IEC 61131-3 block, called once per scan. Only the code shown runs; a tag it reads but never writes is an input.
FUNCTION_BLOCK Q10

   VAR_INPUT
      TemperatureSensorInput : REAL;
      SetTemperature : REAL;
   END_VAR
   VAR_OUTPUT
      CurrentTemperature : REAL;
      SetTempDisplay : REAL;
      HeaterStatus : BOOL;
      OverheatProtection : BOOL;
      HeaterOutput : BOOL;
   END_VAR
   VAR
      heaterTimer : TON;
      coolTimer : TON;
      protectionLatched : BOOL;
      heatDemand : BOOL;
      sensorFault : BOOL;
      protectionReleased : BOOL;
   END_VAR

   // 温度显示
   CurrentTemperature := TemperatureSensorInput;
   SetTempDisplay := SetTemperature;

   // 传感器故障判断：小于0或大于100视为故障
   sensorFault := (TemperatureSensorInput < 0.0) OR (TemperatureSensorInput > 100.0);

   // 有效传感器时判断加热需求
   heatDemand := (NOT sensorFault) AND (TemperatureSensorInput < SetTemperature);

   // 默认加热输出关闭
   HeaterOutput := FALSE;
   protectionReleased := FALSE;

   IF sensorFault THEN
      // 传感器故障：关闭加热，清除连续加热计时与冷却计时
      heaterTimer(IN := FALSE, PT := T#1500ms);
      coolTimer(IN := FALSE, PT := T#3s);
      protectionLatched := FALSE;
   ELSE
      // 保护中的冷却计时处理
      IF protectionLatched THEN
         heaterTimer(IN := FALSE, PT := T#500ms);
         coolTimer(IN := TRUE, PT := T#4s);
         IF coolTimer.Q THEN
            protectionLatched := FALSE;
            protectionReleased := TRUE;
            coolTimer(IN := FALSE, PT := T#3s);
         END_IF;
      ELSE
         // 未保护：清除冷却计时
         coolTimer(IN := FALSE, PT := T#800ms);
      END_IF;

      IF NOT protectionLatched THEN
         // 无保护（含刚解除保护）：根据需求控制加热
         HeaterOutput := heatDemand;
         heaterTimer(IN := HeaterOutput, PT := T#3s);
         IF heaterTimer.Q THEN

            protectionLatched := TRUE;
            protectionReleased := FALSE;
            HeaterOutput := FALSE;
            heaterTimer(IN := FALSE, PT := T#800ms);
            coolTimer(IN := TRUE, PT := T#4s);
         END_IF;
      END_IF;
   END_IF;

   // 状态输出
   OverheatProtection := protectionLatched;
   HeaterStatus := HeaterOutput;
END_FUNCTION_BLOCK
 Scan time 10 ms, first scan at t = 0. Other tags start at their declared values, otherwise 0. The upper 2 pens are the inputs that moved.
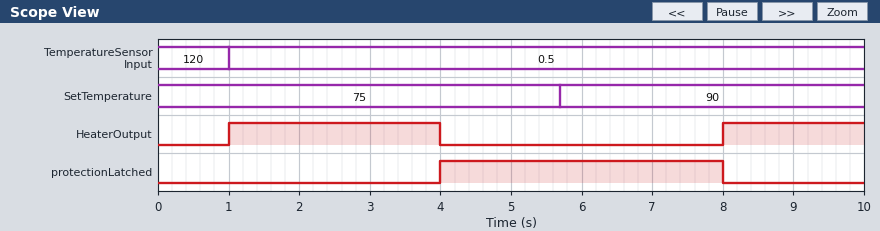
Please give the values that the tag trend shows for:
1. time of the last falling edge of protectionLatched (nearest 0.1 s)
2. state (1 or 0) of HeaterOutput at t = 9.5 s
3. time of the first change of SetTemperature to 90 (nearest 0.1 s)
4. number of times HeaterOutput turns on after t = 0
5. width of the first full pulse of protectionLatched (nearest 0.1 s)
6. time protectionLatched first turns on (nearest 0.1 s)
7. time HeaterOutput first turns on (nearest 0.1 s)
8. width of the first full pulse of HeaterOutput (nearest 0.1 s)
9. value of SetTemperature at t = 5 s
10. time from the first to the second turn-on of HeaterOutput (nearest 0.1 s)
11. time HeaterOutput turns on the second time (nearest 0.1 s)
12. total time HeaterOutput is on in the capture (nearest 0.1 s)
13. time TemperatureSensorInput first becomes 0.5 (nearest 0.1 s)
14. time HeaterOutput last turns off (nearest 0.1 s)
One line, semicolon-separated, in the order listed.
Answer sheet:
8.0 s; 1; 5.7 s; 2; 4.0 s; 4.0 s; 1.0 s; 3.0 s; 75; 7.0 s; 8.0 s; 5.0 s; 1.0 s; 4.0 s
